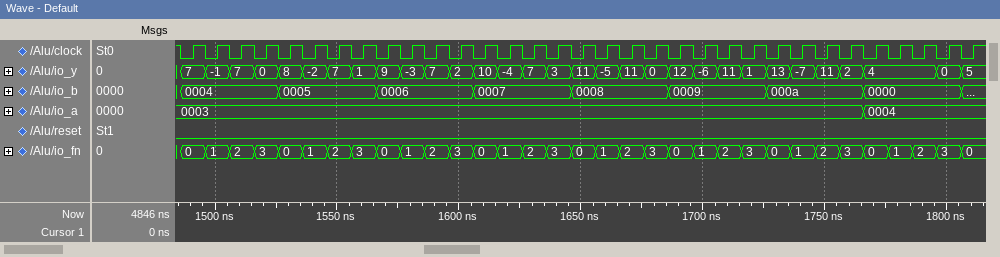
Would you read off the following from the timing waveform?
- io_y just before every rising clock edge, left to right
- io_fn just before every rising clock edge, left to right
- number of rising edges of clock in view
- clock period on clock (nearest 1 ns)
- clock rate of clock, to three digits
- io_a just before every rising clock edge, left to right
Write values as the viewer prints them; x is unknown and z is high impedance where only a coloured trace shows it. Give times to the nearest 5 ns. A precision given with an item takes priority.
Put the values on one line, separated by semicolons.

7, -1, 7, 0, 8, -2, 7, 1, 9, -3, 7, 2, 10, -4, 7, 3, 11, -5, 11, 0, 12, -6, 11, 1, 13, -7, 11, 2, 4, 4, 4, 0, 5; 0, 1, 2, 3, 0, 1, 2, 3, 0, 1, 2, 3, 0, 1, 2, 3, 0, 1, 2, 3, 0, 1, 2, 3, 0, 1, 2, 3, 0, 1, 2, 3, 0; 33; 10 ns; 100 MHz; 0003, 0003, 0003, 0003, 0003, 0003, 0003, 0003, 0003, 0003, 0003, 0003, 0003, 0003, 0003, 0003, 0003, 0003, 0003, 0003, 0003, 0003, 0003, 0003, 0003, 0003, 0003, 0003, 0004, 0004, 0004, 0004, 0004
